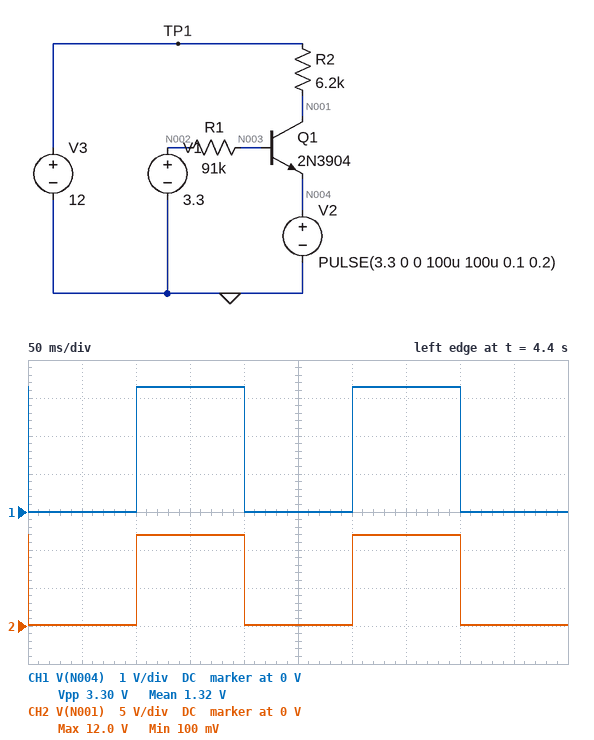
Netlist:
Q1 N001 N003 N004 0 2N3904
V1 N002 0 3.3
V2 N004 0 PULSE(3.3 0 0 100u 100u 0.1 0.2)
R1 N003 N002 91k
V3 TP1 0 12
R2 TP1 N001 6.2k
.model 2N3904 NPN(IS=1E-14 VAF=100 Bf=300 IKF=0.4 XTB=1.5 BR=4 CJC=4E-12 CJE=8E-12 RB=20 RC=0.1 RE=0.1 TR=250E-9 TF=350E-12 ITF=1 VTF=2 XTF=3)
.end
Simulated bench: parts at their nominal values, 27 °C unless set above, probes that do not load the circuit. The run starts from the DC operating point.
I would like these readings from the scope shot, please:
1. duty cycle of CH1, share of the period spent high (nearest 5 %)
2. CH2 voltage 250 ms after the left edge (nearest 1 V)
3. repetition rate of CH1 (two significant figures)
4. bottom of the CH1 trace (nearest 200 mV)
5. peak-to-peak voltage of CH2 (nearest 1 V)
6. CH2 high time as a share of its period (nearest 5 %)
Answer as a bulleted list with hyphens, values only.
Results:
- 50 %
- 0 V
- 5.0 Hz
- 0 V
- 12 V
- 50 %
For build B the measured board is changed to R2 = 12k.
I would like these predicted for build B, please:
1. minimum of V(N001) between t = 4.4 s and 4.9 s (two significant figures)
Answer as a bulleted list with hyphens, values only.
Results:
- 63 mV
